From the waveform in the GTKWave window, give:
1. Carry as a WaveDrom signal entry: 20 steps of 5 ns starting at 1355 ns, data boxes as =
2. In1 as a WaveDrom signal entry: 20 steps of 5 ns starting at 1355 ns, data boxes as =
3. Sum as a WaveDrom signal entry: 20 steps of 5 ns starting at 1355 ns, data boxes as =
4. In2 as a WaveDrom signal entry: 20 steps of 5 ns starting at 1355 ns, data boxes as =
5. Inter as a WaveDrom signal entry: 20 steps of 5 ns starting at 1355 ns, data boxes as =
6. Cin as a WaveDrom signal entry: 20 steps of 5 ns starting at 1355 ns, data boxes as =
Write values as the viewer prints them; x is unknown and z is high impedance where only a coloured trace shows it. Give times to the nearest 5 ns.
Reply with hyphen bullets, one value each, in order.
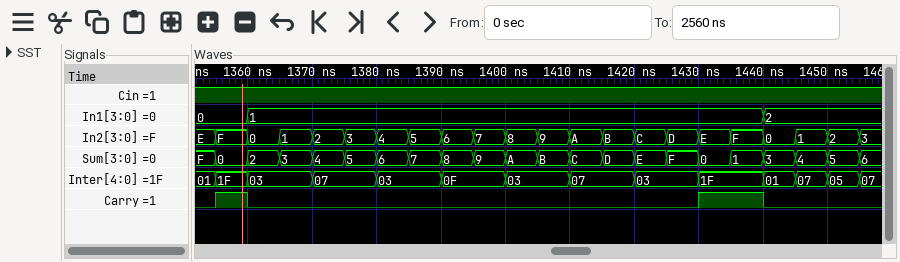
- {name: 'Carry', wave: '10.............1.0..'}
- {name: 'In1', wave: '==...............=..', data: '0 1 2'}
- {name: 'Sum', wave: '====================', data: '0 2 3 4 5 6 7 8 9 A B C D E F 0 1 3 4 5'}
- {name: 'In2', wave: '====================', data: 'F 0 1 2 3 4 5 6 7 8 9 A B C D E F 0 1 2'}
- {name: 'Inter', wave: '==.=.=.=.=.=.=.=.===', data: '1F 03 07 03 0F 03 07 03 1F 01 07 05'}
- {name: 'Cin', wave: '1...................'}
